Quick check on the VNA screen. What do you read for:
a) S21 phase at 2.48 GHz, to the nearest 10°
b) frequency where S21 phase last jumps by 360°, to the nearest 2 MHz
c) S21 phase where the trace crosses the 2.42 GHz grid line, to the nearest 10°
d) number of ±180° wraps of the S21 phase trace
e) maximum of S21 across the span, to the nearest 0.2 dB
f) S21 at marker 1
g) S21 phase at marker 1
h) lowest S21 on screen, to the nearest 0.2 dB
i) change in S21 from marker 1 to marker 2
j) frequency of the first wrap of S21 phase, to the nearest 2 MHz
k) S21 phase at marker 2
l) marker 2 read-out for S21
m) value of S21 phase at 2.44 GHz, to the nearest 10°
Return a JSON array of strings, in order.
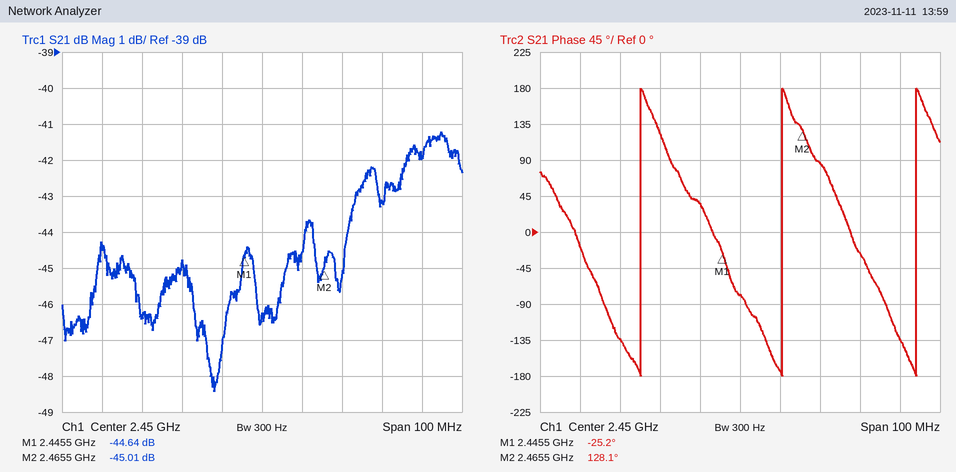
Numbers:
["-30°", "2.494 GHz", "-130°", "3", "-41.2 dB", "-44.64 dB", "-25.2°", "-48.4 dB", "-0.37 dB", "2.426 GHz", "128.1°", "-45.01 dB", "40°"]
